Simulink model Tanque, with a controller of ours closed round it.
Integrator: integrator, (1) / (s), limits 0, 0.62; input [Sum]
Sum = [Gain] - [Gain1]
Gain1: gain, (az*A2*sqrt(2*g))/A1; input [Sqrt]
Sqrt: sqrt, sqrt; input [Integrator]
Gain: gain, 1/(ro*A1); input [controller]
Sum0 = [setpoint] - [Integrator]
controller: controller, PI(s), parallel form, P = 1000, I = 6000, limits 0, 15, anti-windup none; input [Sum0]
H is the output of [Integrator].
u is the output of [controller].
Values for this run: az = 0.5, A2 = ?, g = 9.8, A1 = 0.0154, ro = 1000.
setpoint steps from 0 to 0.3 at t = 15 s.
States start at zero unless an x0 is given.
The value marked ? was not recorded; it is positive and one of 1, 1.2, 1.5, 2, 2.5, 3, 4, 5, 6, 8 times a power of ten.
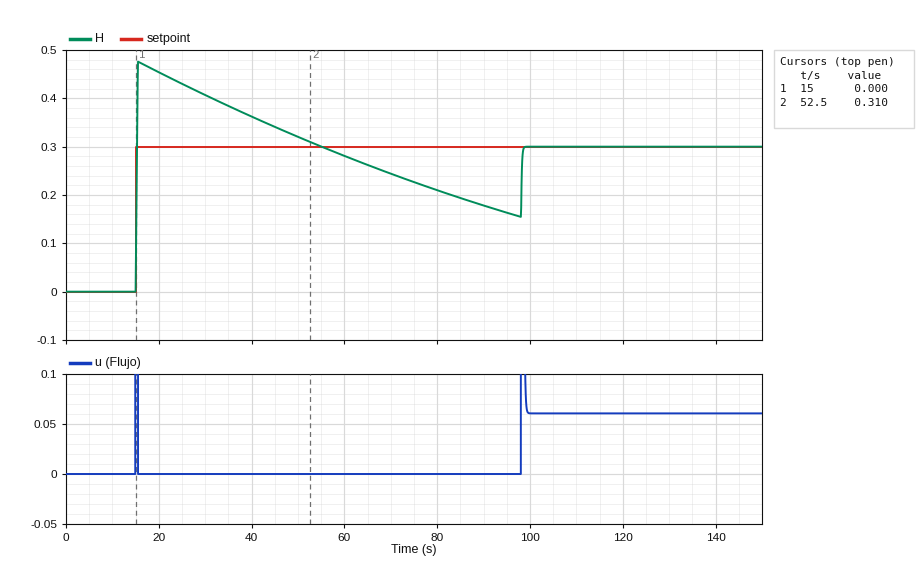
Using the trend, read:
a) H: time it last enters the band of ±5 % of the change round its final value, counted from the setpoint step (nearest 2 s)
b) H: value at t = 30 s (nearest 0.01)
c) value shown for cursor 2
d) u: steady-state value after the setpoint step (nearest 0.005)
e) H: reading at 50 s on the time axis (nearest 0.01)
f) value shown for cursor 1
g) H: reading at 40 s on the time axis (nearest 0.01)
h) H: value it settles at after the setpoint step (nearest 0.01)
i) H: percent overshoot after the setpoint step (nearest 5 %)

84 s
0.41
0.310
0.060
0.32
0.000
0.36
0.30
60 %
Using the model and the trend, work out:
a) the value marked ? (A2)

5e-05
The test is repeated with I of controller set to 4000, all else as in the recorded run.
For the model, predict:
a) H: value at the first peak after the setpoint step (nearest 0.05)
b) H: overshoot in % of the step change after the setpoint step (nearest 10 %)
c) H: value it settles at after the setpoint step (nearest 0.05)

0.45
50 %
0.30
